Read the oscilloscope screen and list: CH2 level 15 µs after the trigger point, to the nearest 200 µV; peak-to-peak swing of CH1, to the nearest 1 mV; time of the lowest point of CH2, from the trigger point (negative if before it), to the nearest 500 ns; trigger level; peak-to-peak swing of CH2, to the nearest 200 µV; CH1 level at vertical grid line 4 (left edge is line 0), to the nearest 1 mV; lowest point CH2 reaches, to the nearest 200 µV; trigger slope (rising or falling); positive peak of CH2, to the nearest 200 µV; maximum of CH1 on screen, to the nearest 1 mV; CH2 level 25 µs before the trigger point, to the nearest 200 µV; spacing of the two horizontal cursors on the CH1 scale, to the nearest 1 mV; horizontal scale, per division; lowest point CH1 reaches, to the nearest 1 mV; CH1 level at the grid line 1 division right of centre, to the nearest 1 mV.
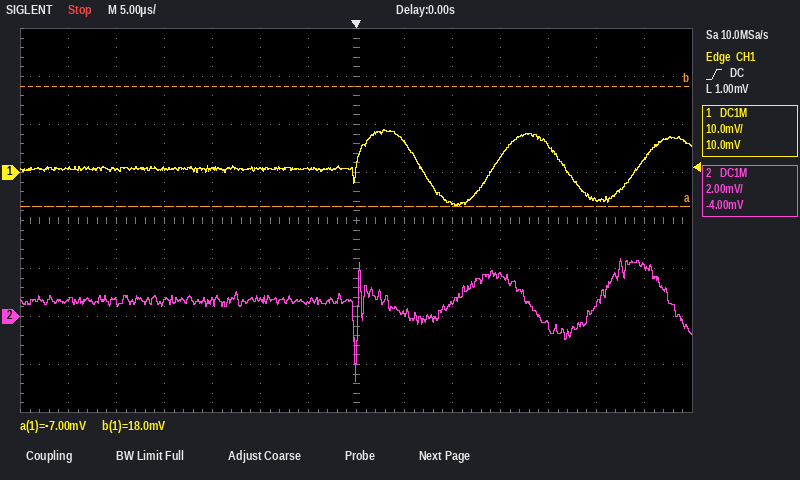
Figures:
1.8 mV
16 mV
0.0 µs
1.00 mV
5.2 mV
1 mV
-2.8 mV
rising
2.4 mV
9 mV
600 µV
25 mV
5 µs
-7 mV
6 mV
